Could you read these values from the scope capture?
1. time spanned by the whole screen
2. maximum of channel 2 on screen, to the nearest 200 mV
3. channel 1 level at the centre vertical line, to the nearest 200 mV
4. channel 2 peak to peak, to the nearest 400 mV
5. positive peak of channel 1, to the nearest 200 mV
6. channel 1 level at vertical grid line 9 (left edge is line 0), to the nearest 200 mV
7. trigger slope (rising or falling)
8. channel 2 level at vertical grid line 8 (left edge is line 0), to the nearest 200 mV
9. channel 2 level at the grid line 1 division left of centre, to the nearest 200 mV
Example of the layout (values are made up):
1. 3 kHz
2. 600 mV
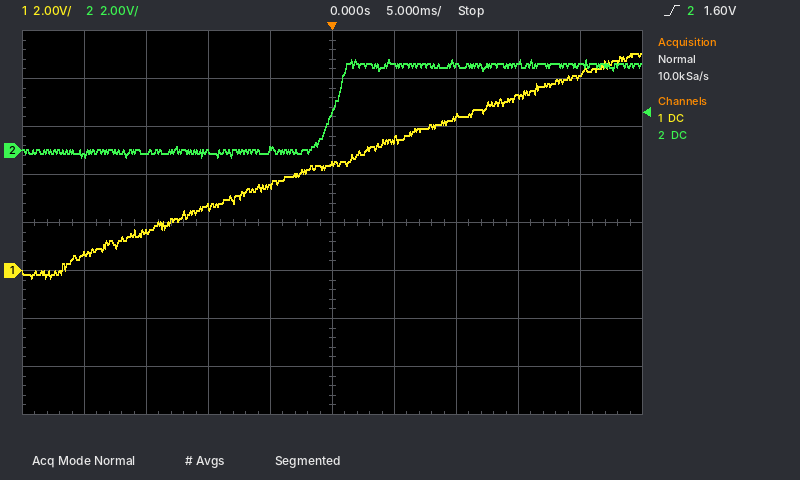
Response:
1. 50 ms
2. 3.8 V
3. 4.4 V
4. 4.0 V
5. 9.0 V
6. 8.2 V
7. rising
8. 3.6 V
9. 0.0 V
